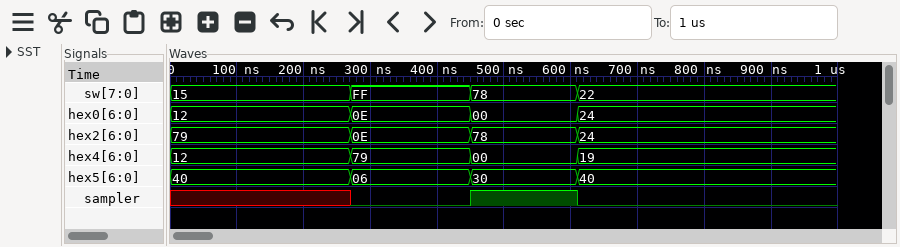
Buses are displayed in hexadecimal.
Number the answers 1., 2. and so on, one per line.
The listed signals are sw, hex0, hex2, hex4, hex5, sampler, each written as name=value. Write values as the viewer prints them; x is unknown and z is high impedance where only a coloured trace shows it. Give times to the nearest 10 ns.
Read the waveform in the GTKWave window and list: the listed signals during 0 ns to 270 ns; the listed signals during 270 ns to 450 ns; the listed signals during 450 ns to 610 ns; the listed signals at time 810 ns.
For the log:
1. sw=15, hex0=12, hex2=79, hex4=12, hex5=40, sampler=x
2. sw=FF, hex0=0E, hex2=0E, hex4=79, hex5=06, sampler=0
3. sw=78, hex0=00, hex2=78, hex4=00, hex5=30, sampler=1
4. sw=22, hex0=24, hex2=24, hex4=19, hex5=40, sampler=0
